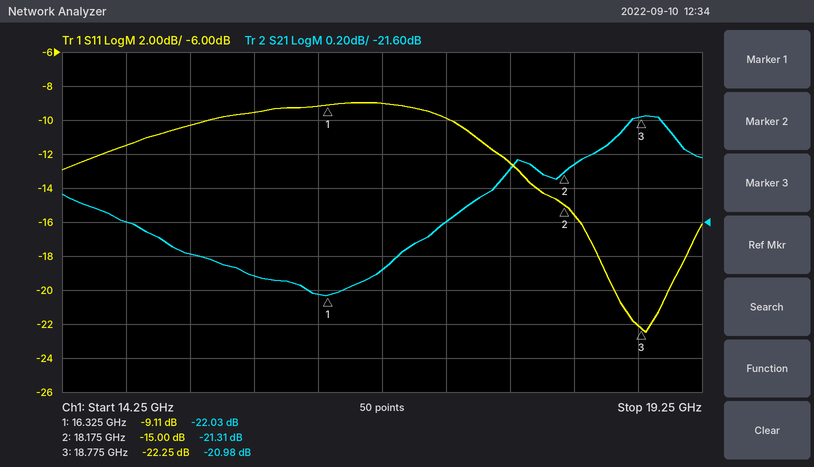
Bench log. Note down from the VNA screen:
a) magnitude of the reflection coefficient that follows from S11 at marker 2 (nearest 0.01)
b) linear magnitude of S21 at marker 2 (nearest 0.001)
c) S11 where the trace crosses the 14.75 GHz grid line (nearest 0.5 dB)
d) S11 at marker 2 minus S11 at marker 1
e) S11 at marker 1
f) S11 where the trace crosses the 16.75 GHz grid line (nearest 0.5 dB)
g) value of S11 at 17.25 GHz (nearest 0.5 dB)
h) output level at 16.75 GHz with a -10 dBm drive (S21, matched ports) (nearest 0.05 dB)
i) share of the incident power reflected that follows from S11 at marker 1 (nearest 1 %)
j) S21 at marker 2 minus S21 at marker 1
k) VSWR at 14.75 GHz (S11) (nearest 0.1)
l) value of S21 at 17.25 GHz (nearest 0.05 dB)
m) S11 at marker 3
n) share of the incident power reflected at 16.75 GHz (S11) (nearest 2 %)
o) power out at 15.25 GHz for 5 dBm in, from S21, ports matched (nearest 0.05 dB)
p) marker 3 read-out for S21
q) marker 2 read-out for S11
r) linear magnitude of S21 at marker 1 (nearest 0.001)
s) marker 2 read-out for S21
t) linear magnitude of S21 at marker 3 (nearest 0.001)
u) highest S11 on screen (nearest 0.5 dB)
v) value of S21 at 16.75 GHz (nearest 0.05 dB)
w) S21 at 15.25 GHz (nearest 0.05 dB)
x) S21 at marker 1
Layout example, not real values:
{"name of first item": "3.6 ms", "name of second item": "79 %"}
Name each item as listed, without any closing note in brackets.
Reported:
{"magnitude of the reflection coefficient that follows from S11 at marker 2": "0.18", "linear magnitude of S21 at marker 2": "0.086", "S11 where the trace crosses the 14.75 GHz grid line": "-11.5 dB", "S11 at marker 2 minus S11 at marker 1": "-5.89 dB", "S11 at marker 1": "-9.11 dB", "S11 where the trace crosses the 16.75 GHz grid line": "-9.0 dB", "value of S11 at 17.25 GHz": "-10.0 dB", "output level at 16.75 GHz with a -10 dBm drive (S21, matched ports)": "-31.90 dBm", "share of the incident power reflected that follows from S11 at marker 1": "12 %", "S21 at marker 2 minus S21 at marker 1": "0.72 dB", "VSWR at 14.75 GHz (S11)": "1.7", "value of S21 at 17.25 GHz": "-21.60 dB", "S11 at marker 3": "-22.25 dB", "share of the incident power reflected at 16.75 GHz (S11)": "12 %", "power out at 15.25 GHz for 5 dBm in, from S21, ports matched": "-16.80 dBm", "marker 3 read-out for S21": "-20.98 dB", "marker 2 read-out for S11": "-15.00 dB", "linear magnitude of S21 at marker 1": "0.079", "marker 2 read-out for S21": "-21.31 dB", "linear magnitude of S21 at marker 3": "0.089", "highest S11 on screen": "-9.0 dB", "value of S21 at 16.75 GHz": "-21.90 dB", "S21 at 15.25 GHz": "-21.80 dB", "S21 at marker 1": "-22.03 dB"}
